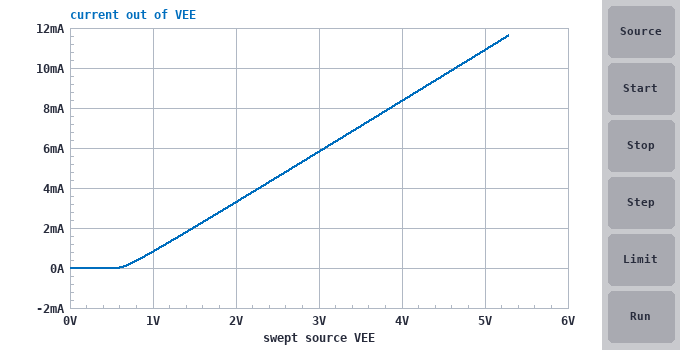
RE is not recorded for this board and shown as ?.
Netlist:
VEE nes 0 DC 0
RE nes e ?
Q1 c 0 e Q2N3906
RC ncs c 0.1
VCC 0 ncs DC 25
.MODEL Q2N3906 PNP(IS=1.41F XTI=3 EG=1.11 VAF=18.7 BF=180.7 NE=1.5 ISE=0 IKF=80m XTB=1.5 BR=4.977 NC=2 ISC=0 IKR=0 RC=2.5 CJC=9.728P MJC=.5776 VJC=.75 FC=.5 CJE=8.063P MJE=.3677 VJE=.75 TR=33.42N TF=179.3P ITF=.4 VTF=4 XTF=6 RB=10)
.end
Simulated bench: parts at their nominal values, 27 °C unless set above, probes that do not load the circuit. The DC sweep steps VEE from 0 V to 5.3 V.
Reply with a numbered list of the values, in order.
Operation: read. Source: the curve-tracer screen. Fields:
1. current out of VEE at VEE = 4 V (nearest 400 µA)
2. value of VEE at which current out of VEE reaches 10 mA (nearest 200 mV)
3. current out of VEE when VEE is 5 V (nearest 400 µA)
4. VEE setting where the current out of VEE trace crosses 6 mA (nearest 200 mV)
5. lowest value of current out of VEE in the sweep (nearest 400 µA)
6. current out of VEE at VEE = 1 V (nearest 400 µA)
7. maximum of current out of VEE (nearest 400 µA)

1. 8.4 mA
2. 4.6 V
3. 10.8 mA
4. 3.0 V
5. 0 A
6. 800 µA
7. 11.6 mA
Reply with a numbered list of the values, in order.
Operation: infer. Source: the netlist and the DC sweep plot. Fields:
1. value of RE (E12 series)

1. 390 Ω
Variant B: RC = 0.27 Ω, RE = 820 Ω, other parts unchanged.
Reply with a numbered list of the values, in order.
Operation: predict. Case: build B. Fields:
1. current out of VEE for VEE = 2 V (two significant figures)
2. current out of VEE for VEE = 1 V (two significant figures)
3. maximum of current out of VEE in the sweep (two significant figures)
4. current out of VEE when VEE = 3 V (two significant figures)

1. 1.6 mA
2. 410 µA
3. 5.6 mA
4. 2.8 mA
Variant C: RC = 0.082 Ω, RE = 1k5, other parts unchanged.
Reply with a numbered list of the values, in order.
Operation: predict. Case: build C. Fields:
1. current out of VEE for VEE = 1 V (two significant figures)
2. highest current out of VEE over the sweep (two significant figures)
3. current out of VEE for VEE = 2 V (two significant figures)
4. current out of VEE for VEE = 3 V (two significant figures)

1. 240 µA
2. 3.1 mA
3. 880 µA
4. 1.5 mA
